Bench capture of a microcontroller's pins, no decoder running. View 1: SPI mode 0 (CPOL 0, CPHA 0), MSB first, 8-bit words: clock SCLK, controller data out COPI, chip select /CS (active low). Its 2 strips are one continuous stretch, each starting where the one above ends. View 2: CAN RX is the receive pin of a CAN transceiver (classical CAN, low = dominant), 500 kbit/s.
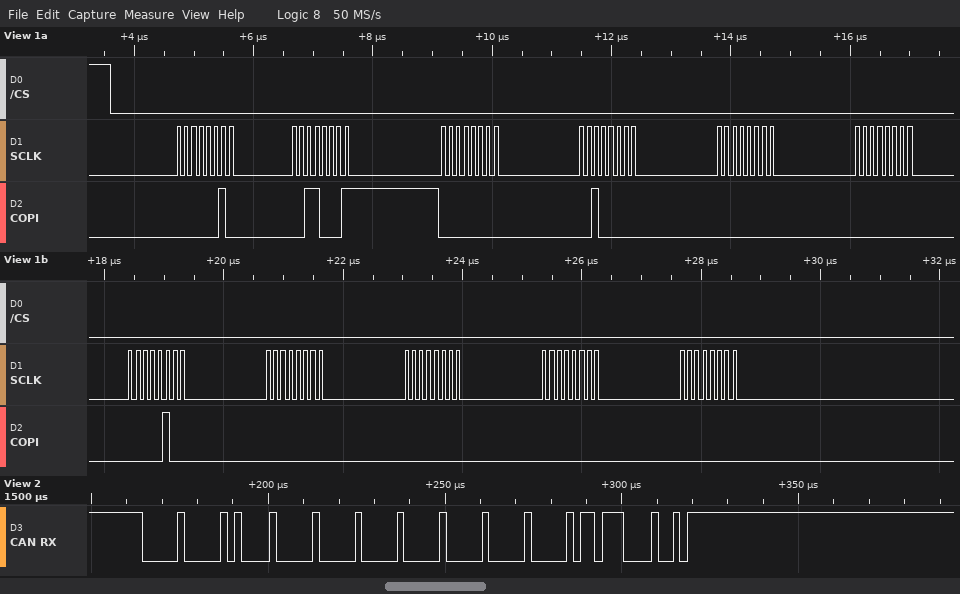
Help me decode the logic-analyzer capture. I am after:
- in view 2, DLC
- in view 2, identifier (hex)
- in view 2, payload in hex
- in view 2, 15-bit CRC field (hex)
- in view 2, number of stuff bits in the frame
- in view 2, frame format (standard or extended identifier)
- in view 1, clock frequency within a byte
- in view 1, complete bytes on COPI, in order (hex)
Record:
4
0x001
00 00 00 00
0x1B84
9
standard
8 MHz
02 31 00 20 00 00 04 00 00 00 00
